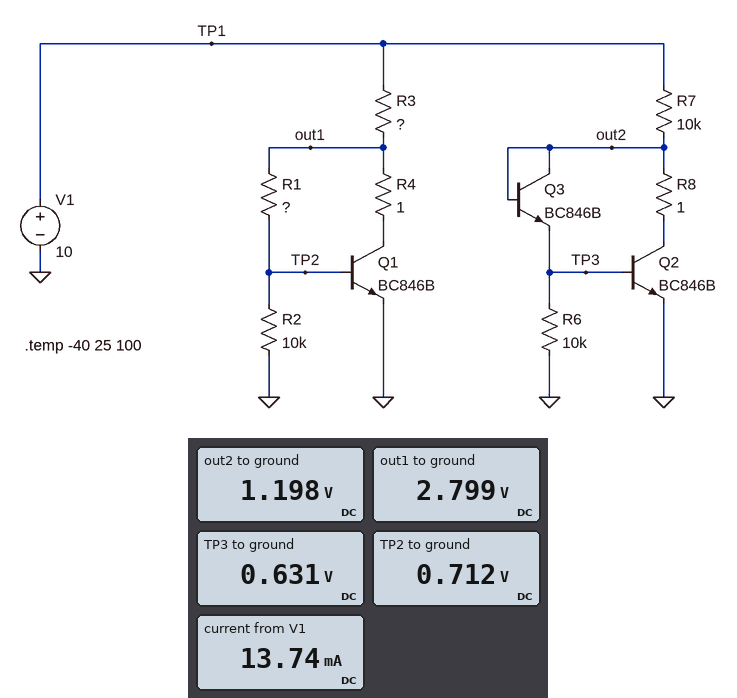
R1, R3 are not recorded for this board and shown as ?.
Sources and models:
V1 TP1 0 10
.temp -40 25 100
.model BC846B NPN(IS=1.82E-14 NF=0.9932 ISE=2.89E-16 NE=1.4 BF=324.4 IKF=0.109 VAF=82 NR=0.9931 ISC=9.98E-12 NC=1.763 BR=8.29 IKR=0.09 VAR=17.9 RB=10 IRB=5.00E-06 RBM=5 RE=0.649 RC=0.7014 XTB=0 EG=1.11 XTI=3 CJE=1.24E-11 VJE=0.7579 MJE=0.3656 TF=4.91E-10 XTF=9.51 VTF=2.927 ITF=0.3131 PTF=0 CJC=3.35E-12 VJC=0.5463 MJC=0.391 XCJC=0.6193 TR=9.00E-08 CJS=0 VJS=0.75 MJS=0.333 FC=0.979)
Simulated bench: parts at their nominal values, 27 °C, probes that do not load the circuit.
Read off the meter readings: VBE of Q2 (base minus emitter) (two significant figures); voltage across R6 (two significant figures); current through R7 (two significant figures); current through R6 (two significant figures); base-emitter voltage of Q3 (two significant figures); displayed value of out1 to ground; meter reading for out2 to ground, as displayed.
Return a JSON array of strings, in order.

["630 mV", "630 mV", "880 µA", "63 µA", "570 mV", "2.799 V", "1.198 V"]
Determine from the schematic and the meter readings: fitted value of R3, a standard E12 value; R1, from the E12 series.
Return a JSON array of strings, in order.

["560 Ω", "18 kΩ"]
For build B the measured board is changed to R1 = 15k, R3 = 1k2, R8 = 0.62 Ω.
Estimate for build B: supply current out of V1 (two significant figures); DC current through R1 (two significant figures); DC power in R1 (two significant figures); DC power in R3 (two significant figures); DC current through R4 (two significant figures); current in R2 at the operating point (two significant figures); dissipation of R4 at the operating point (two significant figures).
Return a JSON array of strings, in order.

["7.5 mA", "91 µA", "120 µW", "53 mW", "6.5 mA", "69 µA", "43 µW"]
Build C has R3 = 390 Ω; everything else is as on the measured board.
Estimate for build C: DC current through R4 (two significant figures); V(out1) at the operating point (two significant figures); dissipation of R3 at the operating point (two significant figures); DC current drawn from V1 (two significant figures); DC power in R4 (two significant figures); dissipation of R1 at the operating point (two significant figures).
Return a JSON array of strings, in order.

["17 mA", "3.2 V", "120 mW", "18 mA", "300 µW", "330 µW"]
